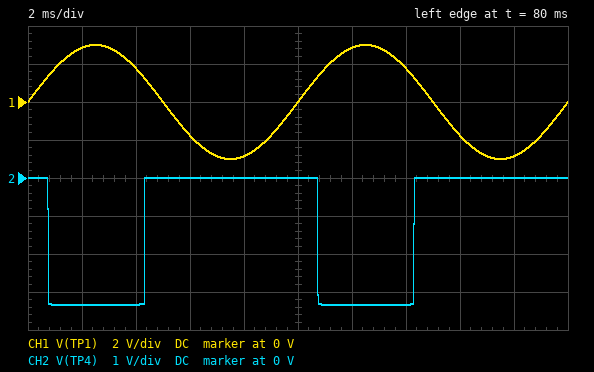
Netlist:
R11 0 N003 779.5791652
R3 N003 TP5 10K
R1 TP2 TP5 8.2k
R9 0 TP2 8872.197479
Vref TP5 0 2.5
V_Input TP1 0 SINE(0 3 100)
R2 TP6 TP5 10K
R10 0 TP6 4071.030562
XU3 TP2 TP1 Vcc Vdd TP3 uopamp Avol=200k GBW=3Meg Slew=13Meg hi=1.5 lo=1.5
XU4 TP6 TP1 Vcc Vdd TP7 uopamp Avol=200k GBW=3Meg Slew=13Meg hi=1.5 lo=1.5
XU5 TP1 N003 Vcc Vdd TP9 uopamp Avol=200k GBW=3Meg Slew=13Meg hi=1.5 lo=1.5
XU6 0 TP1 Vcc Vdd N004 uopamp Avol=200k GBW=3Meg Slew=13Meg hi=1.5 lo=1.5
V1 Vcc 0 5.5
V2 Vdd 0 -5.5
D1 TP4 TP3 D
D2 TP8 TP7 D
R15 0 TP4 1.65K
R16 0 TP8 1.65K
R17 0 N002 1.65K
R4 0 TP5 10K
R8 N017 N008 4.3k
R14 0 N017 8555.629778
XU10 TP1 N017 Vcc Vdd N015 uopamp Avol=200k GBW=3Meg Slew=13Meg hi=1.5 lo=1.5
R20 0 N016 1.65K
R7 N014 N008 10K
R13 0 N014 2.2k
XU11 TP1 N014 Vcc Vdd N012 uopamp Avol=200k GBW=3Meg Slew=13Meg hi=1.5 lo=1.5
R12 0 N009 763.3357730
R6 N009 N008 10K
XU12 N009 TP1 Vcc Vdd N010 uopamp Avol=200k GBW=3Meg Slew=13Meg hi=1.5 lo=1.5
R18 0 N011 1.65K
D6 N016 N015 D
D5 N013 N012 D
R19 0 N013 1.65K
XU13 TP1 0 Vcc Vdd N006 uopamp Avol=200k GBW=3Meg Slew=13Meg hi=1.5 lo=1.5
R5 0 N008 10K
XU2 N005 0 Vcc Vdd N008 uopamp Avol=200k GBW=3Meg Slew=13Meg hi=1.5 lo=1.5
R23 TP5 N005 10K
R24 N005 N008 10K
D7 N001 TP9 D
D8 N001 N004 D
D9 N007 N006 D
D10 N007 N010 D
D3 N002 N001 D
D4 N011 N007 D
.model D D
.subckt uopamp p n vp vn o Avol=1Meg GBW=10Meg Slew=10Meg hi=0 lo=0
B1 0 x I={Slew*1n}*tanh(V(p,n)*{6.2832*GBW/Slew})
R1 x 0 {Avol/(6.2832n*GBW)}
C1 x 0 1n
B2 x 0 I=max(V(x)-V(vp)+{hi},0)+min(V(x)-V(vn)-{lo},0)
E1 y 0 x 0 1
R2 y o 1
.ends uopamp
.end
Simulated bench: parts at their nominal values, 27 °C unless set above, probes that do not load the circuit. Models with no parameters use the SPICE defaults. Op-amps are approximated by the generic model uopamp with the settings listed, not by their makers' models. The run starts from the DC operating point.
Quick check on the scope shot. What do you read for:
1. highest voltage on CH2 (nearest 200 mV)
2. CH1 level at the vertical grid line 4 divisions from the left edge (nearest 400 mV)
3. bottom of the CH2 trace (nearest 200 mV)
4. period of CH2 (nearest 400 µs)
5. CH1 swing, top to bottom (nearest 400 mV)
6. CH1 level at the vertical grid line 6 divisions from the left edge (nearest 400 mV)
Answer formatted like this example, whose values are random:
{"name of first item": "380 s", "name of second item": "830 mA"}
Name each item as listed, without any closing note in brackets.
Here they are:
{"highest voltage on CH2": "0 V", "CH1 level at the vertical grid line 4 divisions from the left edge": "-2.8 V", "bottom of the CH2 trace": "-3.4 V", "period of CH2": "10.0 ms", "CH1 swing, top to bottom": "6.0 V", "CH1 level at the vertical grid line 6 divisions from the left edge": "2.8 V"}
